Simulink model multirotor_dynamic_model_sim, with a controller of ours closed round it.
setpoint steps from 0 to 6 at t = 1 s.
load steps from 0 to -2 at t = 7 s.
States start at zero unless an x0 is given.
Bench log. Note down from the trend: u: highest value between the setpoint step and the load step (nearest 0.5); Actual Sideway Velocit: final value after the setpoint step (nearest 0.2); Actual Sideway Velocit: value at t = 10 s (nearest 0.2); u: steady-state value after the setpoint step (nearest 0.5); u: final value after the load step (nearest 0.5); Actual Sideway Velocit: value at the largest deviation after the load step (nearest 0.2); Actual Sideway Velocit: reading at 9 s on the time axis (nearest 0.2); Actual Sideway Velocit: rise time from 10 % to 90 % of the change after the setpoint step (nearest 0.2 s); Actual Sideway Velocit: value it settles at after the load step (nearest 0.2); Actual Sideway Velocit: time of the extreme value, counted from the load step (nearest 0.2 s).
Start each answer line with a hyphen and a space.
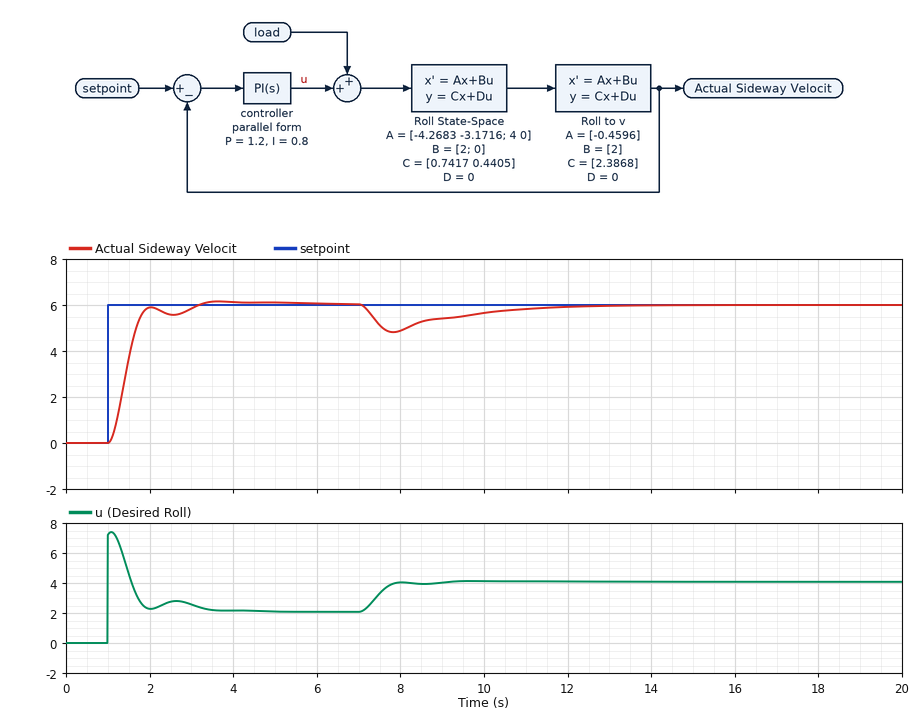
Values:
- 7.5
- 6.0
- 5.6
- 2.0
- 4.0
- 4.8
- 5.4
- 0.6 s
- 6.0
- 0.8 s
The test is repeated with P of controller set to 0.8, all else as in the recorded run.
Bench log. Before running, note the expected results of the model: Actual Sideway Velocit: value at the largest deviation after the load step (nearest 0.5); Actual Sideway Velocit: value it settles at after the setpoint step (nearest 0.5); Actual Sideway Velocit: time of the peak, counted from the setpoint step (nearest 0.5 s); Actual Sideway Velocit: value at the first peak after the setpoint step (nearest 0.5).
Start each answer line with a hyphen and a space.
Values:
- 4.5
- 6.0
- 3.0 s
- 6.5
